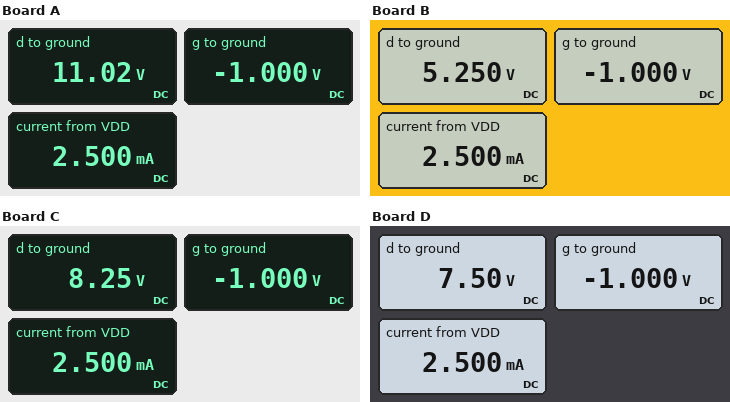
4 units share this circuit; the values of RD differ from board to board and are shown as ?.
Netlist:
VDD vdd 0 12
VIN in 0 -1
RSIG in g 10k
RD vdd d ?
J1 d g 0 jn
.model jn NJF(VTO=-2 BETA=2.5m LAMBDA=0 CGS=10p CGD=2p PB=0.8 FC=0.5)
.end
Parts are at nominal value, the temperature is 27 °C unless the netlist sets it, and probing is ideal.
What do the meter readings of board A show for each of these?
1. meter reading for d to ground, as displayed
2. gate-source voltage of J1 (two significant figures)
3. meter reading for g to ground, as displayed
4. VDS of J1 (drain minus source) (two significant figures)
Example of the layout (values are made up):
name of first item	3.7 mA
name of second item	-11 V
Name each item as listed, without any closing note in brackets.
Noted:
meter reading for d to ground, as displayed	11.02 V
gate-source voltage of J1	-1.0 V
meter reading for g to ground, as displayed	-1.000 V
VDS of J1 (drain minus source)	11 V
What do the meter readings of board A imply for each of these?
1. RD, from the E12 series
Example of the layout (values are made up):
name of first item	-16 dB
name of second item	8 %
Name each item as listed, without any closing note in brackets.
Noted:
RD, from the E12 series	390 Ω
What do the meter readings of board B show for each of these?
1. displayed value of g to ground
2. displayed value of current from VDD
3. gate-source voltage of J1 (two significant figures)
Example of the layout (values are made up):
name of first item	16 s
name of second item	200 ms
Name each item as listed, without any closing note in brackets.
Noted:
displayed value of g to ground	-1.000 V
displayed value of current from VDD	2.500 mA
gate-source voltage of J1	-1.0 V
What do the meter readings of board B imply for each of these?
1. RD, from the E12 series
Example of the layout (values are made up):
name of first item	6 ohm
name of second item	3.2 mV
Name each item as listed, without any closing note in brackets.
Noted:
RD, from the E12 series	2.7 kΩ
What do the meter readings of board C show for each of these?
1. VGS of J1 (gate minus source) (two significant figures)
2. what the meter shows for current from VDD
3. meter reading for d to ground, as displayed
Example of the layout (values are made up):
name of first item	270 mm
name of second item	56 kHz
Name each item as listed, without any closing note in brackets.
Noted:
VGS of J1 (gate minus source)	-1.0 V
what the meter shows for current from VDD	2.500 mA
meter reading for d to ground, as displayed	8.25 V
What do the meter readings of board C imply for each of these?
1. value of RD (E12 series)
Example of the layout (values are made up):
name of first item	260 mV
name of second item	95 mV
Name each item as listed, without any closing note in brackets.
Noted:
value of RD	1.5 kΩ
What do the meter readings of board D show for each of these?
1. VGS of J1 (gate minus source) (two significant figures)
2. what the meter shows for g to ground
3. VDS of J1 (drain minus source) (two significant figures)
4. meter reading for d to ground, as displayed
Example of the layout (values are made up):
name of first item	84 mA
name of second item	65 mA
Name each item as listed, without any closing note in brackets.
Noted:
VGS of J1 (gate minus source)	-1.0 V
what the meter shows for g to ground	-1.000 V
VDS of J1 (drain minus source)	7.5 V
meter reading for d to ground, as displayed	7.50 V
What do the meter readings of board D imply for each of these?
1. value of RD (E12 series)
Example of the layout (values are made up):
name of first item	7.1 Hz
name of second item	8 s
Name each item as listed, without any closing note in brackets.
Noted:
value of RD	1.8 kΩ
